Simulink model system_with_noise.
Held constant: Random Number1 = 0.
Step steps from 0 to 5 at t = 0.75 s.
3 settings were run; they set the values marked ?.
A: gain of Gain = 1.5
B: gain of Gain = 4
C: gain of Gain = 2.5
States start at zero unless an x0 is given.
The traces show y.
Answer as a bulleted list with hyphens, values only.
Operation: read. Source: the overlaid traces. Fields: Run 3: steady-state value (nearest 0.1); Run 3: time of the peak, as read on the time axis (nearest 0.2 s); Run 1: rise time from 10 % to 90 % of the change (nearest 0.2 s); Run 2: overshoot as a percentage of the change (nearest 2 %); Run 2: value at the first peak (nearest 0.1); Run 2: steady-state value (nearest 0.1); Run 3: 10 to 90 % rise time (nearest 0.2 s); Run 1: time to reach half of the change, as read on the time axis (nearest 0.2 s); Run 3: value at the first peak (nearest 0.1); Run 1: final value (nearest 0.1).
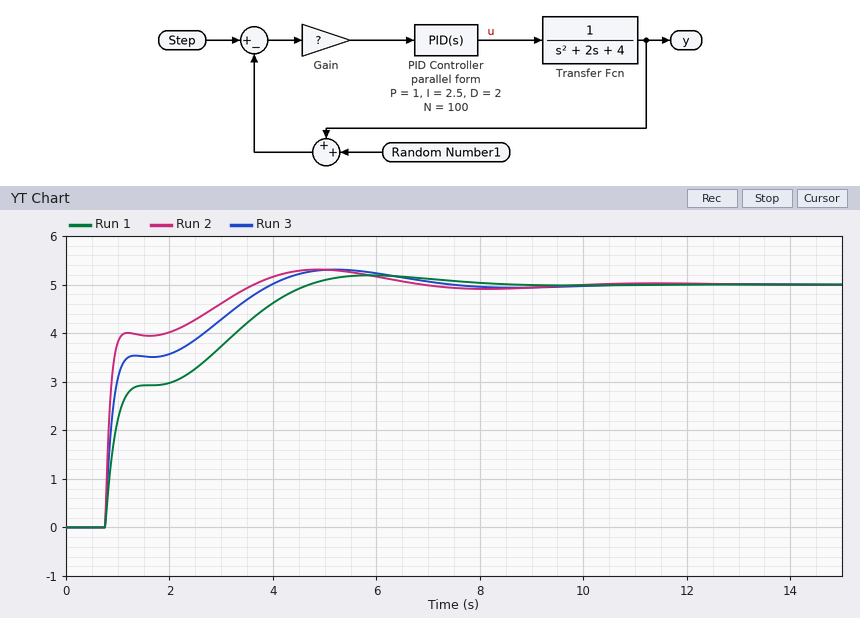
- 5.0
- 5.2 s
- 3.0 s
- 6 %
- 5.3
- 5.0
- 2.4 s
- 1.0 s
- 5.3
- 5.0
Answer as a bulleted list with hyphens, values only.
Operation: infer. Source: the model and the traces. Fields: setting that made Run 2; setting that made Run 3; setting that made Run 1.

- B
- C
- A
